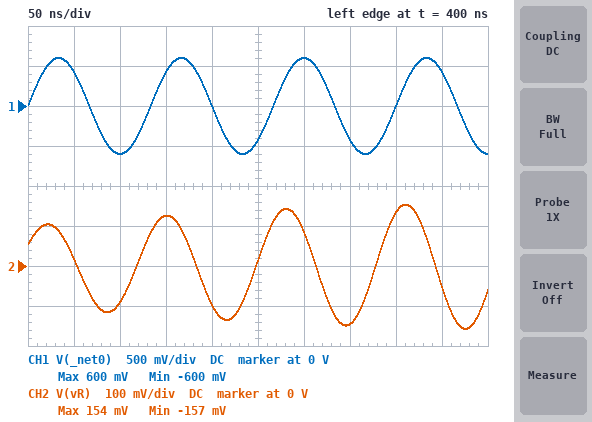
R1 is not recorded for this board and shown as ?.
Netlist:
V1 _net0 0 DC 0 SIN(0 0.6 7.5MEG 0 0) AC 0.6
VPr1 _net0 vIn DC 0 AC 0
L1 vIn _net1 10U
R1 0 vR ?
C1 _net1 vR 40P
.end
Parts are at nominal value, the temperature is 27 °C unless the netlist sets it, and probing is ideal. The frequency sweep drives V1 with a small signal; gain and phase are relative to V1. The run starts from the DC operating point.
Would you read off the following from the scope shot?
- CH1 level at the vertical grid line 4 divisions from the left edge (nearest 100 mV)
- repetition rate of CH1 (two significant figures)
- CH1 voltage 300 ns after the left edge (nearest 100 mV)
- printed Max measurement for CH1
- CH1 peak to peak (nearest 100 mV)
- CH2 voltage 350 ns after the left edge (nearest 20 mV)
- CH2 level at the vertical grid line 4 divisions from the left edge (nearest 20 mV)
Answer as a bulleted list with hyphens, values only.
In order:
- 0 V
- 7.5 MHz
- 600 mV
- 600 mV
- 1.2 V
- -140 mV
- -100 mV
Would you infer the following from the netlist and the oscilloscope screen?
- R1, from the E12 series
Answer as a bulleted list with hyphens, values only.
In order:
- 10 Ω
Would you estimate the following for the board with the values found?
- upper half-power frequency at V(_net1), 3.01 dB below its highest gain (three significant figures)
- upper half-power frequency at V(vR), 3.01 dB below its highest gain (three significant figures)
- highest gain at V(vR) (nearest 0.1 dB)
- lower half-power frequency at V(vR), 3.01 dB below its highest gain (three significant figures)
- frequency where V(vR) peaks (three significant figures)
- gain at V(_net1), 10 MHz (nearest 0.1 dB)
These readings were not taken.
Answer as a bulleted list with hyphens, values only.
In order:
- 8.04 MHz
- 8.04 MHz
- 0 dB
- 7.88 MHz
- 7.96 MHz
- 4.7 dB
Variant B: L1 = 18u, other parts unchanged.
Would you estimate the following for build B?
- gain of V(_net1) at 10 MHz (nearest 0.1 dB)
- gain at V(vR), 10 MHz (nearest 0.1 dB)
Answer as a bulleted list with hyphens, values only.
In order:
- -5.3 dB
- -37.3 dB
